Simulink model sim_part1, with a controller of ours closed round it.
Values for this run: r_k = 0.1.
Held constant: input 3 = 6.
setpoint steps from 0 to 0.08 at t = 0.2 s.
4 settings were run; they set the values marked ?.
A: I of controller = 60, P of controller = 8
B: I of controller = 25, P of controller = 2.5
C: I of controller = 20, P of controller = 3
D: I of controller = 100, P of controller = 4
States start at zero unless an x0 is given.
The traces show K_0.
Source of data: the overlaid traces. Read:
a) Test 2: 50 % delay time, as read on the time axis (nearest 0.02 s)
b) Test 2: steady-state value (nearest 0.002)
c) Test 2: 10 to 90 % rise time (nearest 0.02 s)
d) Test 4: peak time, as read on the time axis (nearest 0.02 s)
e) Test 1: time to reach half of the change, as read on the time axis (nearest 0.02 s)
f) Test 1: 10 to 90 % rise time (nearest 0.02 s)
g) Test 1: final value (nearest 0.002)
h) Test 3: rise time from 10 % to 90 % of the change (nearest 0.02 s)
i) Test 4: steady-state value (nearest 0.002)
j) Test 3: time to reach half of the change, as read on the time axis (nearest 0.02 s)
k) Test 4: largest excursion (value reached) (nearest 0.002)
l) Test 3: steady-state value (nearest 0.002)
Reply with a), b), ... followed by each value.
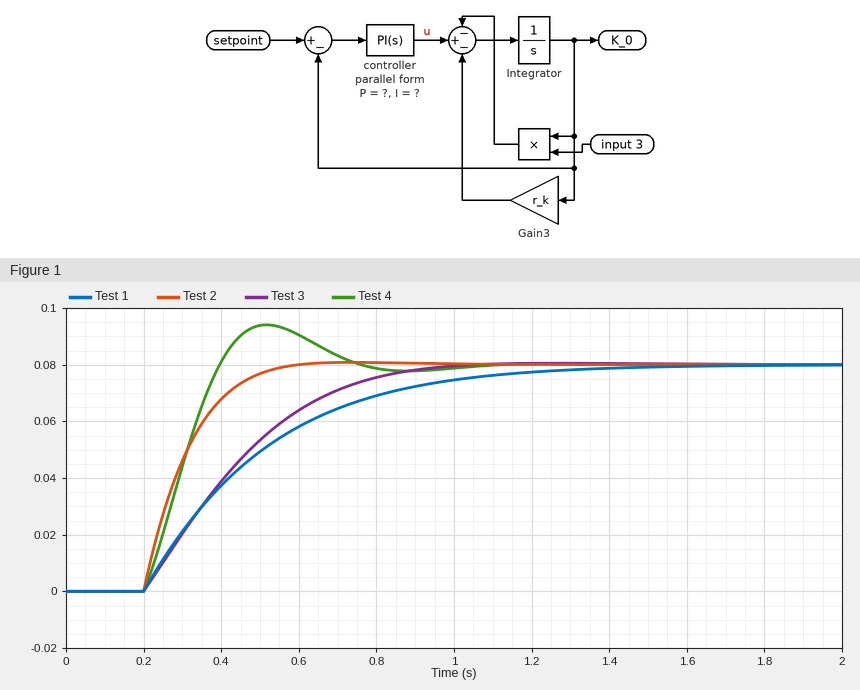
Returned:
a) 0.28 s
b) 0.080
c) 0.22 s
d) 0.52 s
e) 0.42 s
f) 0.66 s
g) 0.080
h) 0.48 s
i) 0.080
j) 0.40 s
k) 0.094
l) 0.080
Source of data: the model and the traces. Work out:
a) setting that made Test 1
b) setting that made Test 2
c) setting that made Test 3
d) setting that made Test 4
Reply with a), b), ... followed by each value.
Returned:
a) C
b) A
c) B
d) D
